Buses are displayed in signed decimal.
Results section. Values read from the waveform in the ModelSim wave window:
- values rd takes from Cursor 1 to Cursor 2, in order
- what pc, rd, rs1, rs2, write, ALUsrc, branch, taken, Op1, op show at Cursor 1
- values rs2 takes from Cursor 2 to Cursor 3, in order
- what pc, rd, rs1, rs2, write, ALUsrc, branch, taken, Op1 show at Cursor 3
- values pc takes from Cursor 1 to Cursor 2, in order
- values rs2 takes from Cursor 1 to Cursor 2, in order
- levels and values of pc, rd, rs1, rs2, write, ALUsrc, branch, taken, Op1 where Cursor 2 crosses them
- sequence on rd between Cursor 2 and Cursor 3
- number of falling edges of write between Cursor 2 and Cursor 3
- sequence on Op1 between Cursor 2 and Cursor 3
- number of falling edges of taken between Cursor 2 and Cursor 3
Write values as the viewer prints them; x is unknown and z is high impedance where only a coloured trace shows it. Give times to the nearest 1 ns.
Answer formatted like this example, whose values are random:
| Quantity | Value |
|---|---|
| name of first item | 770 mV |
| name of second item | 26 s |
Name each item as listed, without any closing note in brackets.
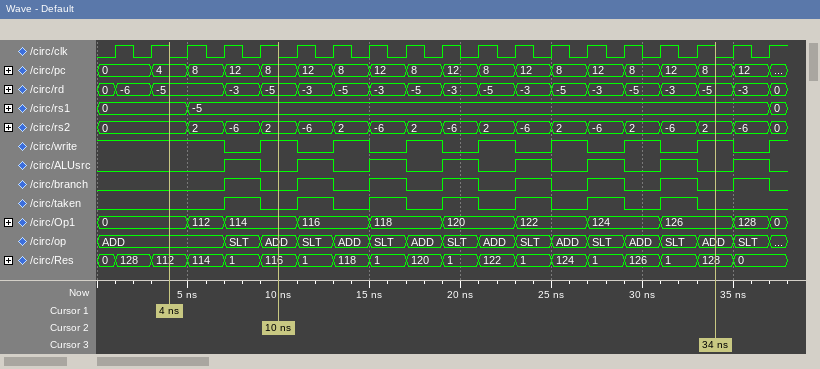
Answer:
| Quantity | Value |
|---|---|
| values rd takes from Cursor 1 to Cursor 2, in order | -5, -3, -5 |
| what pc, rd, rs1, rs2, write, ALUsrc, branch, taken, Op1, op show at Cursor 1 | pc=4, rd=-5, rs1=0, rs2=0, write=1, ALUsrc=0, branch=0, taken=0, Op1=0, op=ADD |
| values rs2 takes from Cursor 2 to Cursor 3, in order | 2, -6, 2, -6, 2, -6, 2, -6, 2, -6, 2, -6, 2 |
| what pc, rd, rs1, rs2, write, ALUsrc, branch, taken, Op1 show at Cursor 3 | pc=8, rd=-5, rs1=-5, rs2=2, write=1, ALUsrc=0, branch=0, taken=0, Op1=126 |
| values pc takes from Cursor 1 to Cursor 2, in order | 4, 8, 12, 8 |
| values rs2 takes from Cursor 1 to Cursor 2, in order | 0, 2, -6, 2 |
| levels and values of pc, rd, rs1, rs2, write, ALUsrc, branch, taken, Op1 where Cursor 2 crosses them | pc=8, rd=-5, rs1=-5, rs2=2, write=1, ALUsrc=0, branch=0, taken=0, Op1=114 |
| sequence on rd between Cursor 2 and Cursor 3 | -5, -3, -5, -3, -5, -3, -5, -3, -5, -3, -5, -3, -5 |
| number of falling edges of write between Cursor 2 and Cursor 3 | 6 |
| sequence on Op1 between Cursor 2 and Cursor 3 | 114, 116, 118, 120, 122, 124, 126 |
| number of falling edges of taken between Cursor 2 and Cursor 3 | 6 |
